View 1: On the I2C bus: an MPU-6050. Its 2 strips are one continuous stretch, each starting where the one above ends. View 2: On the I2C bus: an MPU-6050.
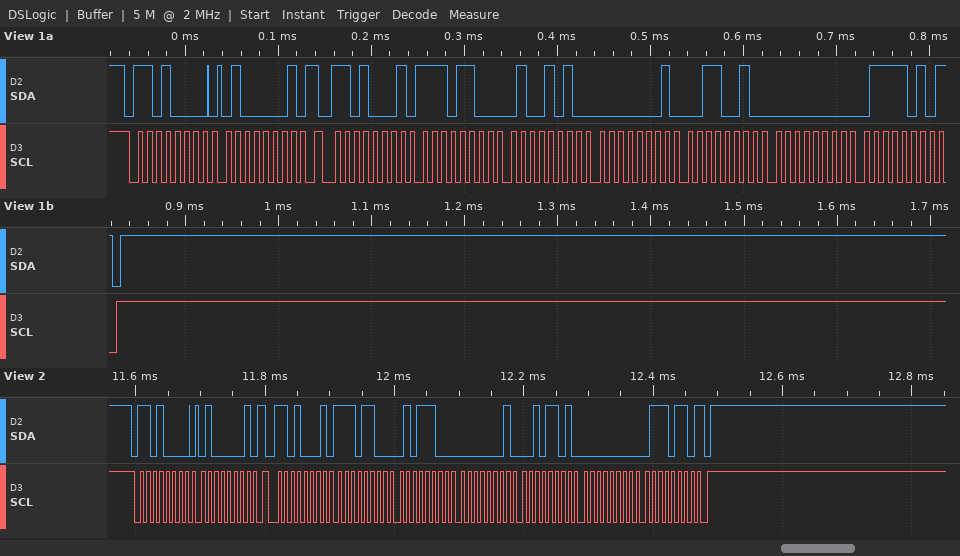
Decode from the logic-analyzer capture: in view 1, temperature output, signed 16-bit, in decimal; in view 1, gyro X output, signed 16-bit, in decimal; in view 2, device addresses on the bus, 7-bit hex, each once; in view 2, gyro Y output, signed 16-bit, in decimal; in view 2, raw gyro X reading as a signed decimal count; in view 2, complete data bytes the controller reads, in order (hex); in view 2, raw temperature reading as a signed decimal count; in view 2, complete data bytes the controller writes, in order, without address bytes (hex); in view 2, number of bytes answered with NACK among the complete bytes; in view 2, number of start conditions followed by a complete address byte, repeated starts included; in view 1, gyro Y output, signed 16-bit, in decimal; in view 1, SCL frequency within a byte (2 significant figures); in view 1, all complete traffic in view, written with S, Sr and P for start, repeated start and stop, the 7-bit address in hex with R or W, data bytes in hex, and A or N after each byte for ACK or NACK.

-5046
306
0x68
118
301
EC 5C 01 2D 00 76
-5028
41
1
2
122
100 kHz
S 68W A 41 A Sr 68R A EC A 4A A 01 A 32 A 00 A 7A N P
